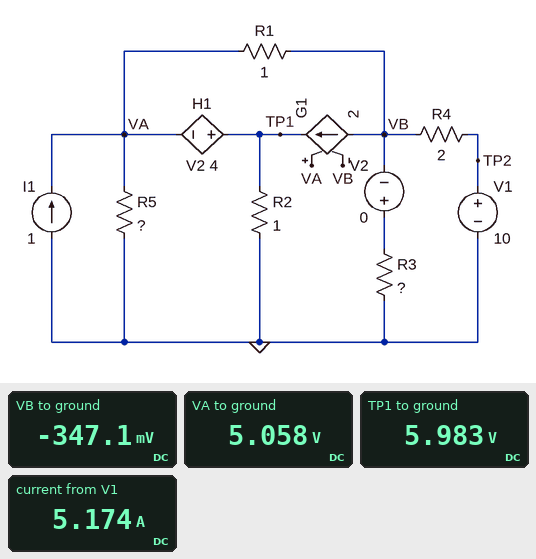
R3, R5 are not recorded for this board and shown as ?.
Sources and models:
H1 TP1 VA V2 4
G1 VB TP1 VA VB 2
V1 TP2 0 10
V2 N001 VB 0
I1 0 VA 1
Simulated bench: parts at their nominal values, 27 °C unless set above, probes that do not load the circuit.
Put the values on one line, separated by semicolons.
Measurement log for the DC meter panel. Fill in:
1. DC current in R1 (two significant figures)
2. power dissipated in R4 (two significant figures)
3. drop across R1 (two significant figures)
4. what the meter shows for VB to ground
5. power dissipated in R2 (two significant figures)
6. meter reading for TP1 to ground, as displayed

5.4 A; 54 W; 5.4 V; -347.1 mV; 36 W; 5.983 V
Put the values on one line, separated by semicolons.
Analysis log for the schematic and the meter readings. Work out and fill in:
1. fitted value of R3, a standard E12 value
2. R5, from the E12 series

1.5 Ω; 12 Ω
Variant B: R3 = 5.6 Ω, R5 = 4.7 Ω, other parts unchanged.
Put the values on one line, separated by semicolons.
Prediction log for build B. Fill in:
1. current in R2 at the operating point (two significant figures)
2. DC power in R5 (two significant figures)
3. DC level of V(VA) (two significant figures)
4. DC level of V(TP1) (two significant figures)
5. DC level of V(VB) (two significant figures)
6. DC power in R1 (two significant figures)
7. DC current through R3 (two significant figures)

5.1 A; 5.2 W; 4.9 V; 5.1 V; -180 mV; 26 W; 32 mA
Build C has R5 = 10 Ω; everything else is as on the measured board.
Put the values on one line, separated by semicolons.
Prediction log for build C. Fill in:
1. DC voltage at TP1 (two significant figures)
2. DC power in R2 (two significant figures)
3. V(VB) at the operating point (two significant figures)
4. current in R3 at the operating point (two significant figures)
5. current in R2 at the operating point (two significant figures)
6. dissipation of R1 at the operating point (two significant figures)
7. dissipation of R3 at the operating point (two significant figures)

5.8 V; 34 W; -300 mV; 200 mA; 5.8 A; 29 W; 59 mW
